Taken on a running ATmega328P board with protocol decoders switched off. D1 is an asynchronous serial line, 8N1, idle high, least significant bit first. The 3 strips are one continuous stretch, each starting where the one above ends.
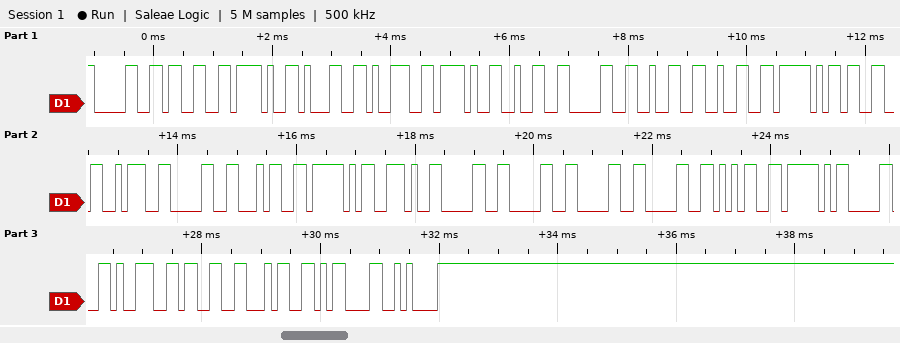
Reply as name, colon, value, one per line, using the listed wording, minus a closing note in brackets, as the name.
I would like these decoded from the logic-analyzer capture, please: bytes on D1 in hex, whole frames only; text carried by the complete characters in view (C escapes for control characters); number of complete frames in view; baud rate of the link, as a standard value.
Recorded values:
bytes on D1 in hex, whole frames only: 30 33 2F 31 39 2F 32 30 32 32 5F 33 3A 30 34 5F 2E 30 30 30 30 35 5F 30 39 33 34 0D 0A
text carried by the complete characters in view: "03/19/2022_3:04_.00005_0934\r\n"
number of complete frames in view: 29
baud rate of the link, as a standard value: 9600 baud
